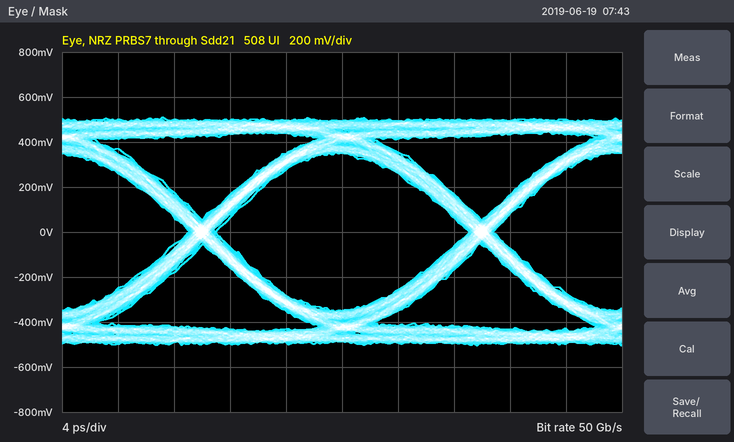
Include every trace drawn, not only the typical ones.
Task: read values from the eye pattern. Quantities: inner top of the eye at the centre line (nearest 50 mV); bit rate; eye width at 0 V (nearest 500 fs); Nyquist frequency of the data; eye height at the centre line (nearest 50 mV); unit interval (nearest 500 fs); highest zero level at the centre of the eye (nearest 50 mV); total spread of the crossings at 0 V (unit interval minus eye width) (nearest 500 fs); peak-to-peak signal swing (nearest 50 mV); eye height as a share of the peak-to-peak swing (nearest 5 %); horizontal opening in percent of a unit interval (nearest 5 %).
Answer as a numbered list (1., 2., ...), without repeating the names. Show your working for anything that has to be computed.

1. 350 mV
2. 50 Gb/s
3. 18.0 ps
4. 25 GHz
5. 700 mV
6. 20.0 ps
7. -350 mV
8. 2.0 ps
9. 1.00 V
10. 700 mV / 1.00 V ≈ 70 %
11. 18.0 ps / 20.0 ps ≈ 90 %
